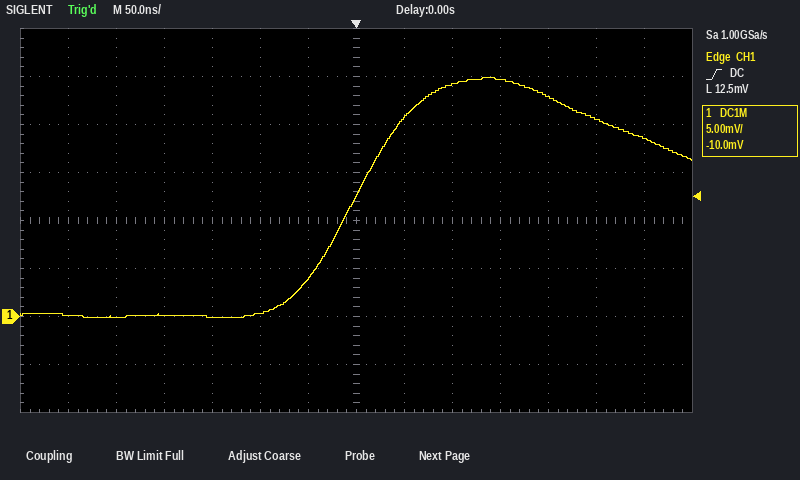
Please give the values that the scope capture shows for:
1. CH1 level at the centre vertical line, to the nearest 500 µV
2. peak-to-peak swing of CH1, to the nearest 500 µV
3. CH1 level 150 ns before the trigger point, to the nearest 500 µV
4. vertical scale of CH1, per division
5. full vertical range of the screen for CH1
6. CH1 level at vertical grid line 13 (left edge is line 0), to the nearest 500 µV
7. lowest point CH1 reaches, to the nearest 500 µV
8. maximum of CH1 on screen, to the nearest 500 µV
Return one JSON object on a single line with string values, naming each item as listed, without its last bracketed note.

{"CH1 level at the centre vertical line, to the nearest 500 µV": "12.5 mV", "peak-to-peak swing of CH1, to the nearest 500 µV": "25.0 mV", "CH1 level 150 ns before the trigger point, to the nearest 500 µV": "0.0 mV", "vertical scale of CH1, per division": "5 mV", "full vertical range of the screen for CH1": "40 mV", "CH1 level at vertical grid line 13 (left edge is line 0), to the nearest 500 µV": "18.5 mV", "lowest point CH1 reaches, to the nearest 500 µV": "0.0 mV", "maximum of CH1 on screen, to the nearest 500 µV": "25.0 mV"}
